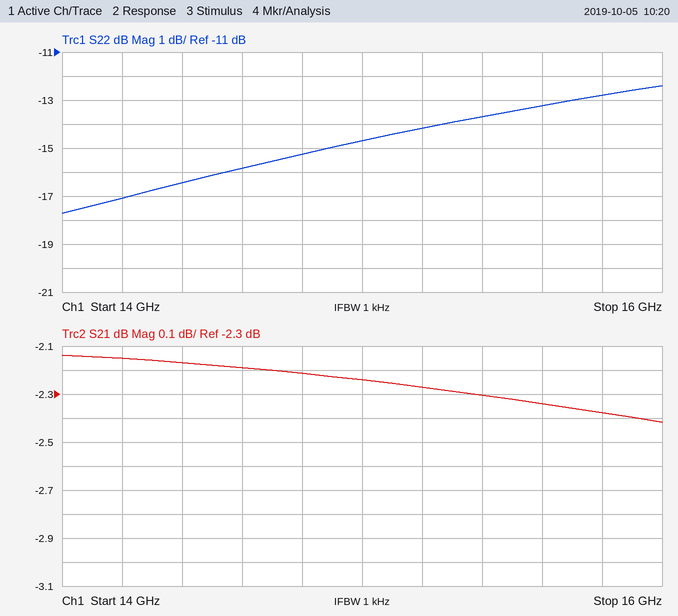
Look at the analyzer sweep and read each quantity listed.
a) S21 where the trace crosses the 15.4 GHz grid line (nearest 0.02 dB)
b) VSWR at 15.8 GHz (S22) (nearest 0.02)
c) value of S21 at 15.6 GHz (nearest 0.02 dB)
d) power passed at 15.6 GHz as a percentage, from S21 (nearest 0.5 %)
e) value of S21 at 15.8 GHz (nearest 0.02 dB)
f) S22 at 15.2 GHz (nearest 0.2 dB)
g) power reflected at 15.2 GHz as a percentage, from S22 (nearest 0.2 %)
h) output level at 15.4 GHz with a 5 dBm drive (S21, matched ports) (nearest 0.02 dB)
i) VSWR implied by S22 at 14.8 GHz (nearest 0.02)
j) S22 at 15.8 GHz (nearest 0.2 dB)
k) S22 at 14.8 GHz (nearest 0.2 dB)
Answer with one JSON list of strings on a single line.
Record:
["-2.30 dB", "1.60", "-2.34 dB", "58.5 %", "-2.38 dB", "-14.2 dB", "3.8 %", "2.70 dBm", "1.42", "-12.8 dB", "-15.2 dB"]
